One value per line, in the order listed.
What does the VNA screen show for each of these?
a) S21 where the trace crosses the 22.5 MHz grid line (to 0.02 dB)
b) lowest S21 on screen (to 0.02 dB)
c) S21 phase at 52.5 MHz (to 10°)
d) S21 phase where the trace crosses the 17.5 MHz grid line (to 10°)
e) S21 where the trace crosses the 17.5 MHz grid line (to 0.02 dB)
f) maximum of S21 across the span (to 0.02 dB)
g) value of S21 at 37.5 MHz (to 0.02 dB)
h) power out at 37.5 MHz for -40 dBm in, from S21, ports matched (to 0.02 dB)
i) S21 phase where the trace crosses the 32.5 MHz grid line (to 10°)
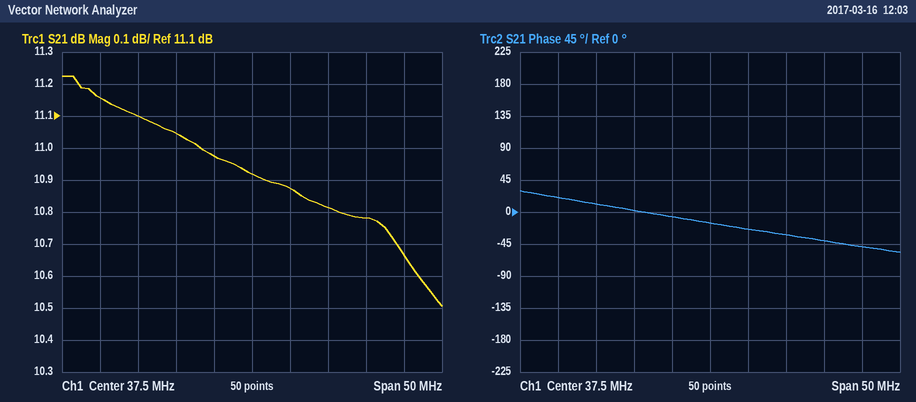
11.10 dB
10.50 dB
-40°
20°
11.16 dB
11.22 dB
10.92 dB
-29.08 dBm
-10°
